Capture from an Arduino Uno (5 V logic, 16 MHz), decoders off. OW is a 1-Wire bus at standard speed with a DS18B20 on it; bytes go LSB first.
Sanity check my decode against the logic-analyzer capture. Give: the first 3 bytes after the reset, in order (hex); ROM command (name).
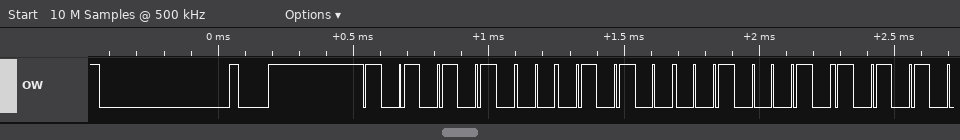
55 28 44
Match ROM
